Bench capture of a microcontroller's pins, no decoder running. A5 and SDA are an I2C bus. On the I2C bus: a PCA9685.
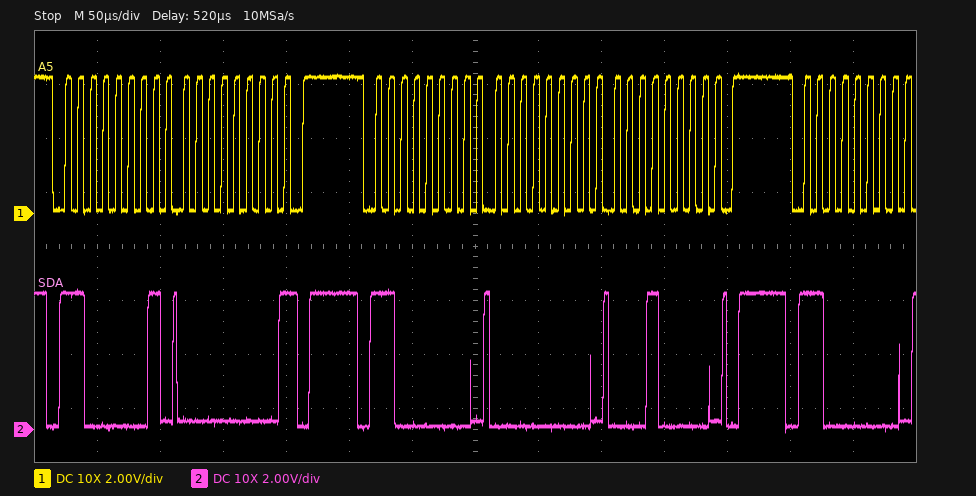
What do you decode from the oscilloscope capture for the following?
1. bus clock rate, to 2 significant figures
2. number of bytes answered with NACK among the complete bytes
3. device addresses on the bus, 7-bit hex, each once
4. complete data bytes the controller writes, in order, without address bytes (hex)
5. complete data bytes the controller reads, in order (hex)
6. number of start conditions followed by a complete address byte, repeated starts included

100 kHz
1
0x60
00 10
00
3
